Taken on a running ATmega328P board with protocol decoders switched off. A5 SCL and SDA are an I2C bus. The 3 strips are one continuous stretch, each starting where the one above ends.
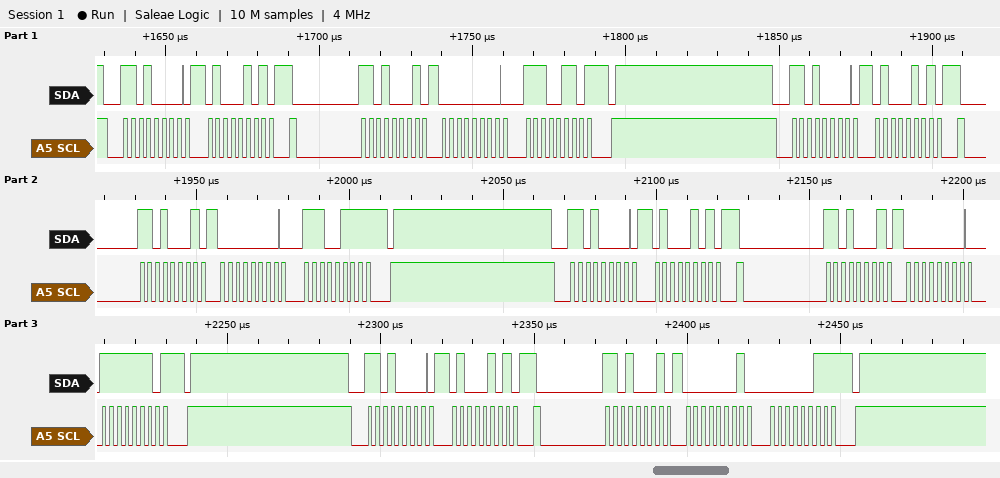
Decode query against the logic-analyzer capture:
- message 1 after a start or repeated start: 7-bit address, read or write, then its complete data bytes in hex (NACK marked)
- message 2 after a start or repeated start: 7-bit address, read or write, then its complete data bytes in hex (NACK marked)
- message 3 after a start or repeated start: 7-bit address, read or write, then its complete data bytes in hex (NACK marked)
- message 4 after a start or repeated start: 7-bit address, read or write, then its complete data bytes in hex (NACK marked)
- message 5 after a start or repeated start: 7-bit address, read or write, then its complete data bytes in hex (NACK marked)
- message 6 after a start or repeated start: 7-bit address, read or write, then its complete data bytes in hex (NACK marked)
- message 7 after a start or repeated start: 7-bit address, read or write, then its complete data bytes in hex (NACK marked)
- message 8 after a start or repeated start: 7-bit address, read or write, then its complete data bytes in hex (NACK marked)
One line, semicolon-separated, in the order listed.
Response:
0x68 write: 45; 0x68 read: 00 E6 NACK; 0x68 write: 45; 0x68 read: 00 E7 NACK; 0x68 write: 45; 0x68 read: 00 FE NACK; 0x68 write: 45; 0x68 read: 01 03 NACK
